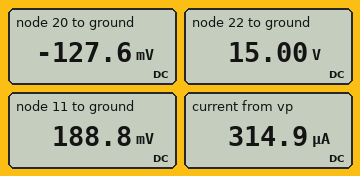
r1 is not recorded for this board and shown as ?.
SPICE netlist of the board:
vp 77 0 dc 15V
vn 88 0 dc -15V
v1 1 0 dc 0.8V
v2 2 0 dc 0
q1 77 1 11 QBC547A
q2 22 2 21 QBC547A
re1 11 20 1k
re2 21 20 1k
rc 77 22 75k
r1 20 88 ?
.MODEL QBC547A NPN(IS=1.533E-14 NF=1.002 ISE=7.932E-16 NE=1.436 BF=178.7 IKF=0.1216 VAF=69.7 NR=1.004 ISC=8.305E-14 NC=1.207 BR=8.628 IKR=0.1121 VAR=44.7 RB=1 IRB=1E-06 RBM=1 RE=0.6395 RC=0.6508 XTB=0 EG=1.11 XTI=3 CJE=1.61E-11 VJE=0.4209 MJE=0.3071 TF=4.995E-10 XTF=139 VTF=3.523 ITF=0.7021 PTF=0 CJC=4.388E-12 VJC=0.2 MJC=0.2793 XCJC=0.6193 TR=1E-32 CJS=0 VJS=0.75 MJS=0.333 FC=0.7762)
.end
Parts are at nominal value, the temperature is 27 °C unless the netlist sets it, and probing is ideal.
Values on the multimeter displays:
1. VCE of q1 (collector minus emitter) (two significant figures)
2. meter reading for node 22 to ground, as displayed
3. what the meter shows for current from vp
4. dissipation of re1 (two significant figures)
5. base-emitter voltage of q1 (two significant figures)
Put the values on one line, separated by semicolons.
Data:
15 V; 15.00 V; 314.9 µA; 100 µW; 610 mV
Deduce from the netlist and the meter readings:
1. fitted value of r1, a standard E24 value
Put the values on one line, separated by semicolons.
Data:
47 kΩ
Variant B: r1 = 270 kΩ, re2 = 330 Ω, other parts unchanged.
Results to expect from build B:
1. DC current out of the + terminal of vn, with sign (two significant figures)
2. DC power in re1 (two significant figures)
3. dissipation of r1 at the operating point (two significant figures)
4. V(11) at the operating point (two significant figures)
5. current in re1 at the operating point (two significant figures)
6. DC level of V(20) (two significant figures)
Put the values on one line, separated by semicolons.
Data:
-56 µA; 3.2 µW; 850 µW; 230 mV; 56 µA; 180 mV
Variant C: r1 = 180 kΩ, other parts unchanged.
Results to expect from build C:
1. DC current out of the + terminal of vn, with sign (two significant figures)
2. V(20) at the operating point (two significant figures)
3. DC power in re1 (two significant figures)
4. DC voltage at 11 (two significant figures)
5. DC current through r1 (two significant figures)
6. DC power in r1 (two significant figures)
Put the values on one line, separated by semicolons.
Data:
-84 µA; 140 mV; 7.1 µW; 220 mV; 84 µA; 1.3 mW
